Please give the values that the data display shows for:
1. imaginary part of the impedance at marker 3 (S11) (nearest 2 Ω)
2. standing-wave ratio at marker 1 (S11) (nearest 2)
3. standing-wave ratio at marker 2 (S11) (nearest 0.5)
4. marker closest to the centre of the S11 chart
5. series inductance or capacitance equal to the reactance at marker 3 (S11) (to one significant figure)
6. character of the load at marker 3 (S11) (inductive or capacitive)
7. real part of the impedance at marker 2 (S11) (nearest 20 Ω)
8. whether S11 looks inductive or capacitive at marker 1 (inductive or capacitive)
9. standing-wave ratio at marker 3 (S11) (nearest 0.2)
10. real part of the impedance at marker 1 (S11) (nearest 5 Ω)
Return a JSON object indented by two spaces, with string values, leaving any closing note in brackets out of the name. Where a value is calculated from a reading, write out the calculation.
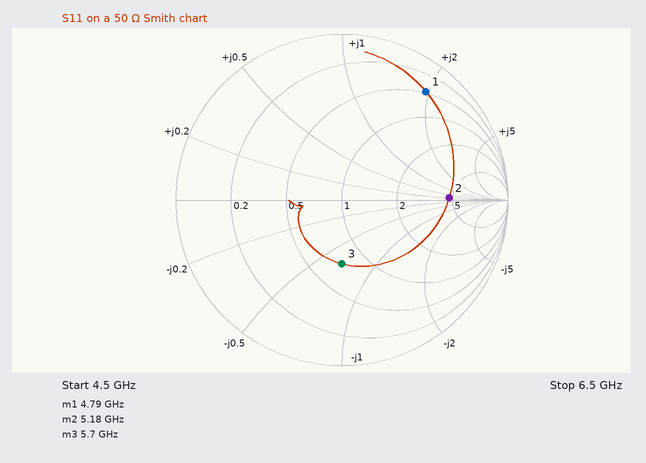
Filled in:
{
  "imaginary part of the impedance at marker 3 (S11)": "-34 Ω",
  "standing-wave ratio at marker 1 (S11)": "10",
  "standing-wave ratio at marker 2 (S11)": "4.5",
  "marker closest to the centre of the S11 chart": "marker 3",
  "series inductance or capacitance equal to the reactance at marker 3 (S11)": "C = 1/(2π × 5.7 GHz × 34 Ω) ≈ 821 fF, so 800 fF to one significant figure",
  "character of the load at marker 3 (S11)": "capacitive",
  "real part of the impedance at marker 2 (S11)": "240 Ω",
  "whether S11 looks inductive or capacitive at marker 1": "inductive",
  "standing-wave ratio at marker 3 (S11)": "2.2",
  "real part of the impedance at marker 1 (S11)": "25 Ω"
}
